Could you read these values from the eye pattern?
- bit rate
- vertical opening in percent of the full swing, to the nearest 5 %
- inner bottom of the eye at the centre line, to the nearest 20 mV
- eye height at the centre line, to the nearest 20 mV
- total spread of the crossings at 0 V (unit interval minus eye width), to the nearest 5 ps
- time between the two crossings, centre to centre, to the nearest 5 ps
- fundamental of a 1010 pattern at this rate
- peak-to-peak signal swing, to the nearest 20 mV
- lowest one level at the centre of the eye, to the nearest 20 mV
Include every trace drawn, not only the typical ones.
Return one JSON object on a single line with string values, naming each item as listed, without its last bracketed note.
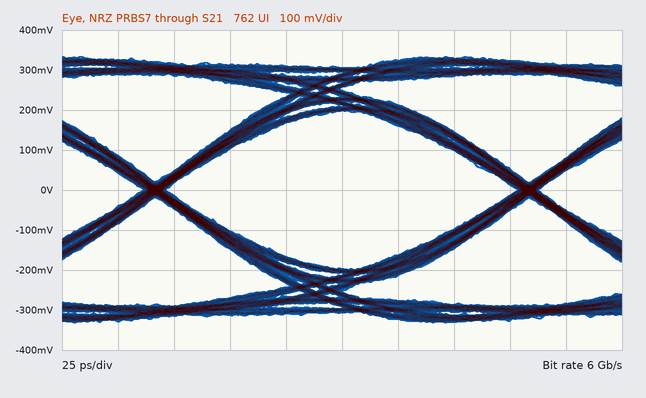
{"bit rate": "6 Gb/s", "vertical opening in percent of the full swing, to the nearest 5 %": "60 %", "inner bottom of the eye at the centre line, to the nearest 20 mV": "-200 mV", "eye height at the centre line, to the nearest 20 mV": "400 mV", "total spread of the crossings at 0 V (unit interval minus eye width), to the nearest 5 ps": "10 ps", "time between the two crossings, centre to centre, to the nearest 5 ps": "165 ps", "fundamental of a 1010 pattern at this rate": "3 GHz", "peak-to-peak signal swing, to the nearest 20 mV": "660 mV", "lowest one level at the centre of the eye, to the nearest 20 mV": "200 mV"}
